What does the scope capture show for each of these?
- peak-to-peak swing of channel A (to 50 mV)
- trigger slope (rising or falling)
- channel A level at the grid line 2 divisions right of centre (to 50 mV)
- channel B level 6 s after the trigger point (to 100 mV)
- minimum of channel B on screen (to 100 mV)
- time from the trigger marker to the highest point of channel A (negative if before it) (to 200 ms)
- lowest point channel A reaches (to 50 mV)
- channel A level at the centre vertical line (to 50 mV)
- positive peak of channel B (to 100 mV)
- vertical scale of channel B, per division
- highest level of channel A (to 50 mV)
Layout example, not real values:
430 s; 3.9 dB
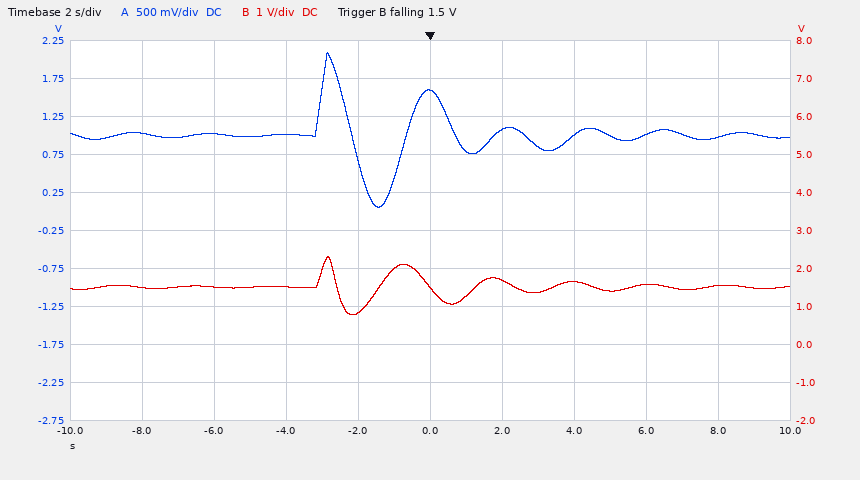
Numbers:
2.05 V; falling; 1.00 V; 1.6 V; 800 mV; -2.8 s; 50 mV; 1.60 V; 2.3 V; 1 V; 2.10 V
